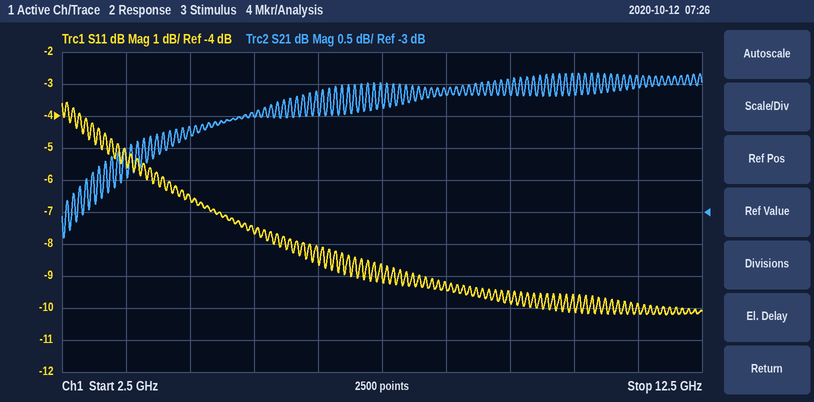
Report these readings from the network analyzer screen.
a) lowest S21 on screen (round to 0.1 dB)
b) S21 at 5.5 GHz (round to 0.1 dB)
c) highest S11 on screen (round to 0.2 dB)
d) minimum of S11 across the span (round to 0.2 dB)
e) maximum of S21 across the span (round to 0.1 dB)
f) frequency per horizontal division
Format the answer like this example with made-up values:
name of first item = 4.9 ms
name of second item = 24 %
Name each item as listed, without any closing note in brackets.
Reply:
lowest S21 on screen = -3.4 dB
S21 at 5.5 GHz = -1.5 dB
highest S11 on screen = -3.6 dB
minimum of S11 across the span = -10.2 dB
maximum of S21 across the span = -0.8 dB
frequency per horizontal division = 1 GHz
